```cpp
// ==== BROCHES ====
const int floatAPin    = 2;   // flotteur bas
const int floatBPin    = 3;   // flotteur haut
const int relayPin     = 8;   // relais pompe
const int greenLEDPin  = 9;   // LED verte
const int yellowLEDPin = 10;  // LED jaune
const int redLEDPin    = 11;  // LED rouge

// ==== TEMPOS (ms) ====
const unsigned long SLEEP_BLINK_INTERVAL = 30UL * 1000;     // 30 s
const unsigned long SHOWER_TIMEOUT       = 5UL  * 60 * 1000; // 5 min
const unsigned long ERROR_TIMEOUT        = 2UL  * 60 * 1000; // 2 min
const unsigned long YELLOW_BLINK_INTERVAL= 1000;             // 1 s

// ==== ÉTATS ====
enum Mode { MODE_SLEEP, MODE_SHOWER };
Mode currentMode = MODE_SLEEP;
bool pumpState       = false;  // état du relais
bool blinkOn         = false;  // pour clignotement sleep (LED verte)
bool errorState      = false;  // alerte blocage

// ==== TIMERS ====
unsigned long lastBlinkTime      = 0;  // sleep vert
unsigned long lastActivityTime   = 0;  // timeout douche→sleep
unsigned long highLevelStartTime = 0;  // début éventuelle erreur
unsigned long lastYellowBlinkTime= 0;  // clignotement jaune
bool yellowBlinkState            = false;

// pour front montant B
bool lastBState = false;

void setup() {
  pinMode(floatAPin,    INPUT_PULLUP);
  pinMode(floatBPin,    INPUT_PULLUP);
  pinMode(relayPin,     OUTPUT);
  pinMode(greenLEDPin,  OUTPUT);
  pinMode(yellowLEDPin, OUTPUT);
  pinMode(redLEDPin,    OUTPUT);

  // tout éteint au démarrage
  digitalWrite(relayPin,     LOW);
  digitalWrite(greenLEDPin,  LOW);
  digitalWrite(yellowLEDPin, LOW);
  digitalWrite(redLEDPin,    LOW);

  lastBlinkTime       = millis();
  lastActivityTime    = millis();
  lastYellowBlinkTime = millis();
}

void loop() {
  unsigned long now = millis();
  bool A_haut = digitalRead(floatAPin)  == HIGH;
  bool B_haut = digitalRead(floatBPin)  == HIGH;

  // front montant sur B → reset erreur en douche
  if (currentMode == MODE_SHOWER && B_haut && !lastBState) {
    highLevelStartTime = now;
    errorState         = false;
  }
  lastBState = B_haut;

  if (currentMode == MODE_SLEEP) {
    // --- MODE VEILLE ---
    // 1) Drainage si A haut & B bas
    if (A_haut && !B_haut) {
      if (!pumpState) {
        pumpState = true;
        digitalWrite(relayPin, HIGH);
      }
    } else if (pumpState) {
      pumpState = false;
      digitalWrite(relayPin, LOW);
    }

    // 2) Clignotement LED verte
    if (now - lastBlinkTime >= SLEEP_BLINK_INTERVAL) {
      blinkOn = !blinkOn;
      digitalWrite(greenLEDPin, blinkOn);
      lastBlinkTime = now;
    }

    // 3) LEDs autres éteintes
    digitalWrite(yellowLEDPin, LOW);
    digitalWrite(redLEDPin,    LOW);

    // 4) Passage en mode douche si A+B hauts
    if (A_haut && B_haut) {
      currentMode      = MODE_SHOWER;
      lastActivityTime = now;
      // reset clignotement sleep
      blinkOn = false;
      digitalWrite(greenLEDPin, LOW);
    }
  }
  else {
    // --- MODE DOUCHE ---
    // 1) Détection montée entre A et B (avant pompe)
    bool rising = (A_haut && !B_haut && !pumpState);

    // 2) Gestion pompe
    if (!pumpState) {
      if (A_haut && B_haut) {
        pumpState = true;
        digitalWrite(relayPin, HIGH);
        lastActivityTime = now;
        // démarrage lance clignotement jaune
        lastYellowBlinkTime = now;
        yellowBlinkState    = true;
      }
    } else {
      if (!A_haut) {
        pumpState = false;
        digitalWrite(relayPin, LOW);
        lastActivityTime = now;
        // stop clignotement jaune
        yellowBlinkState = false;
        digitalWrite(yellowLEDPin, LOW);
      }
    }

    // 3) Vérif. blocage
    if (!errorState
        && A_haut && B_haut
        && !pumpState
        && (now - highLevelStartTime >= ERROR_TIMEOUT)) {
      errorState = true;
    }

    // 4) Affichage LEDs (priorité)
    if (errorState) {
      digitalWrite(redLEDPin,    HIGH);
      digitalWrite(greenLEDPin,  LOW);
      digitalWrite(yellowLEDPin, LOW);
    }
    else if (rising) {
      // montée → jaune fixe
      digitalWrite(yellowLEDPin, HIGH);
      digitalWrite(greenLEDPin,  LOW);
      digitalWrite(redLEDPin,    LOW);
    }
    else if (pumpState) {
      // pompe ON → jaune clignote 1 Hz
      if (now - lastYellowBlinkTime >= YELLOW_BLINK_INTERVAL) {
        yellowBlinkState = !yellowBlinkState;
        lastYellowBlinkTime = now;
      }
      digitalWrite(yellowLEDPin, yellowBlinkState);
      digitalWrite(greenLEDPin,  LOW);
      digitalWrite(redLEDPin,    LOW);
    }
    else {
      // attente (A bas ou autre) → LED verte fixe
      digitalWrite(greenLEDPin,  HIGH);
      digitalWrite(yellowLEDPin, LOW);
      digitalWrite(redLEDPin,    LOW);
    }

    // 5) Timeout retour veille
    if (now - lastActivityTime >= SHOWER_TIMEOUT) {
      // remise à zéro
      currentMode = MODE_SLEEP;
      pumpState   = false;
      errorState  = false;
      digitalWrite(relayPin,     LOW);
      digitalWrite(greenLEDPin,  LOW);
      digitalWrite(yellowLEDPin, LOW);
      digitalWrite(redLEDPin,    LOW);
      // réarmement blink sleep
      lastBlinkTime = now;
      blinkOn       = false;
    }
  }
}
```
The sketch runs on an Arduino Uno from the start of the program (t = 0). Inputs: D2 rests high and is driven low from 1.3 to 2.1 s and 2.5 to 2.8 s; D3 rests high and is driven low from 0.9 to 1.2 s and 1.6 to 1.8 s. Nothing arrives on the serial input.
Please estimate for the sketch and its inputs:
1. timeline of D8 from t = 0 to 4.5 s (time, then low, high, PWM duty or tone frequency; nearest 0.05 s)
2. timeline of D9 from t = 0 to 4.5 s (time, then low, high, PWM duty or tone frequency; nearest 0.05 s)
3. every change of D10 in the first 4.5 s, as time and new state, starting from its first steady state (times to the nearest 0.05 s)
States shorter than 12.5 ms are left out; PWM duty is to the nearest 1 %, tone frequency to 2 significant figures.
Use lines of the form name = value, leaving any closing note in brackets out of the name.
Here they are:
timeline of D8 from t = 0 to 4.5 s = 0 s high; 1.3 s low; 2.1 s high; 2.5 s low; 2.8 s high
timeline of D9 from t = 0 to 4.5 s = 0 s low; 1.3 s high; 2.1 s low; 2.5 s high; 2.8 s low
every change of D10 in the first 4.5 s, as time and new state, starting from its first steady state = 0 s high; 1 s low; 2.1 s high; 2.5 s low; 2.8 s high; 3.8 s low
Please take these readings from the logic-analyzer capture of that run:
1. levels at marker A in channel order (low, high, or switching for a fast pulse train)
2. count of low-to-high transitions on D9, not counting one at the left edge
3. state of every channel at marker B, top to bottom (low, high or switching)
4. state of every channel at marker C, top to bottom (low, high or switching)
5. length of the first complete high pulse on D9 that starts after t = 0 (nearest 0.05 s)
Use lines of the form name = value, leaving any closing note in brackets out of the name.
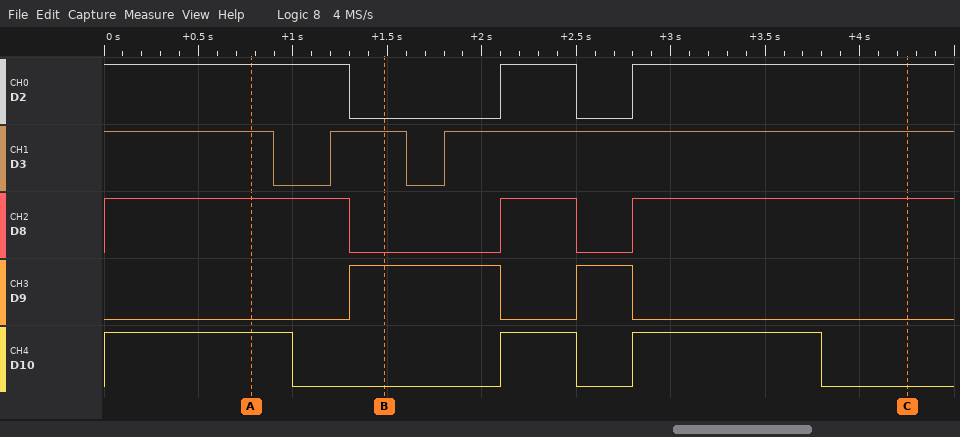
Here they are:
levels at marker A in channel order = D2 high, D3 high, D8 high, D9 low, D10 high
count of low-to-high transitions on D9, not counting one at the left edge = 2
state of every channel at marker B, top to bottom = D2 low, D3 high, D8 low, D9 high, D10 low
state of every channel at marker C, top to bottom = D2 high, D3 high, D8 high, D9 low, D10 low
length of the first complete high pulse on D9 that starts after t = 0 = 0.80 s
